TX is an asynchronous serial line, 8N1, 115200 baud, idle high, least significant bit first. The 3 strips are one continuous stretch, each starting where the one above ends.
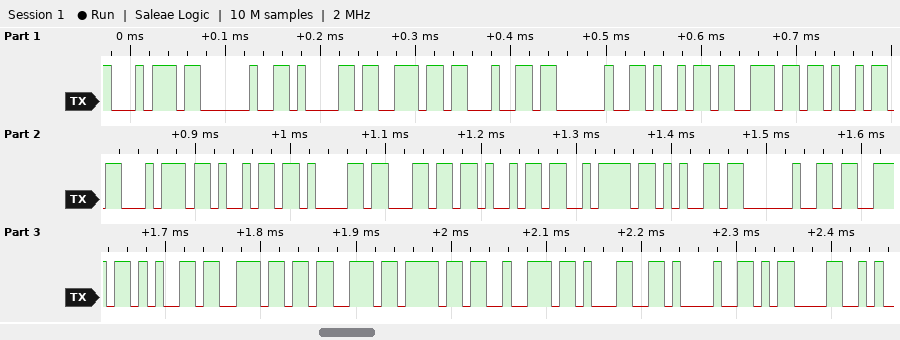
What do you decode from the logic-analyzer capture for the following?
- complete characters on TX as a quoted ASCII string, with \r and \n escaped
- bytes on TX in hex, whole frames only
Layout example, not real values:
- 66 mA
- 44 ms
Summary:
- "t and initialize sensor1!\r"
- 0x74 0x20 0x61 0x6E 0x64 0x20 0x69 0x6E 0x69 0x74 0x69 0x61 0x6C 0x69 0x7A 0x65 0x20 0x73 0x65 0x6E 0x73 0x6F 0x72 0x31 0x21 0x0D
